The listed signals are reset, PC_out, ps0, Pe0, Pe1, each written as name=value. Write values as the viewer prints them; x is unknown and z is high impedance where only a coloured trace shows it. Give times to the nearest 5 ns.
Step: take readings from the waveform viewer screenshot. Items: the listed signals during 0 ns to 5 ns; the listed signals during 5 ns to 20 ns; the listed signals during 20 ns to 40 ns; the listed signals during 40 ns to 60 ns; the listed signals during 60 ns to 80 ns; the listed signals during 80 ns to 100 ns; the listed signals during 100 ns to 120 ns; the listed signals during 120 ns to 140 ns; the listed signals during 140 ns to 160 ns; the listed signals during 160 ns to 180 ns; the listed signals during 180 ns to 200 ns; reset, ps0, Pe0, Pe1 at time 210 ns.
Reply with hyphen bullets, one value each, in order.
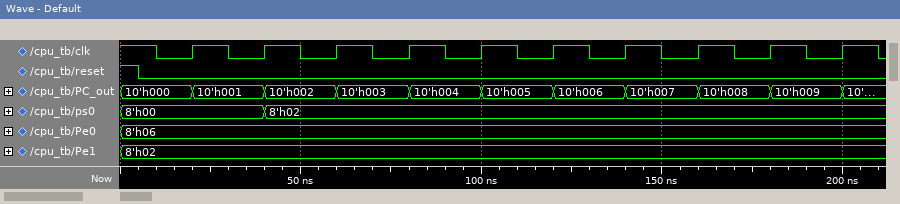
- reset=1, PC_out=10'h000, ps0=8'h00, Pe0=8'h06, Pe1=8'h02
- reset=0, PC_out=10'h000, ps0=8'h00, Pe0=8'h06, Pe1=8'h02
- reset=0, PC_out=10'h001, ps0=8'h00, Pe0=8'h06, Pe1=8'h02
- reset=0, PC_out=10'h002, ps0=8'h02, Pe0=8'h06, Pe1=8'h02
- reset=0, PC_out=10'h003, ps0=8'h02, Pe0=8'h06, Pe1=8'h02
- reset=0, PC_out=10'h004, ps0=8'h02, Pe0=8'h06, Pe1=8'h02
- reset=0, PC_out=10'h005, ps0=8'h02, Pe0=8'h06, Pe1=8'h02
- reset=0, PC_out=10'h006, ps0=8'h02, Pe0=8'h06, Pe1=8'h02
- reset=0, PC_out=10'h007, ps0=8'h02, Pe0=8'h06, Pe1=8'h02
- reset=0, PC_out=10'h008, ps0=8'h02, Pe0=8'h06, Pe1=8'h02
- reset=0, PC_out=10'h009, ps0=8'h02, Pe0=8'h06, Pe1=8'h02
- reset=0, ps0=8'h02, Pe0=8'h06, Pe1=8'h02
